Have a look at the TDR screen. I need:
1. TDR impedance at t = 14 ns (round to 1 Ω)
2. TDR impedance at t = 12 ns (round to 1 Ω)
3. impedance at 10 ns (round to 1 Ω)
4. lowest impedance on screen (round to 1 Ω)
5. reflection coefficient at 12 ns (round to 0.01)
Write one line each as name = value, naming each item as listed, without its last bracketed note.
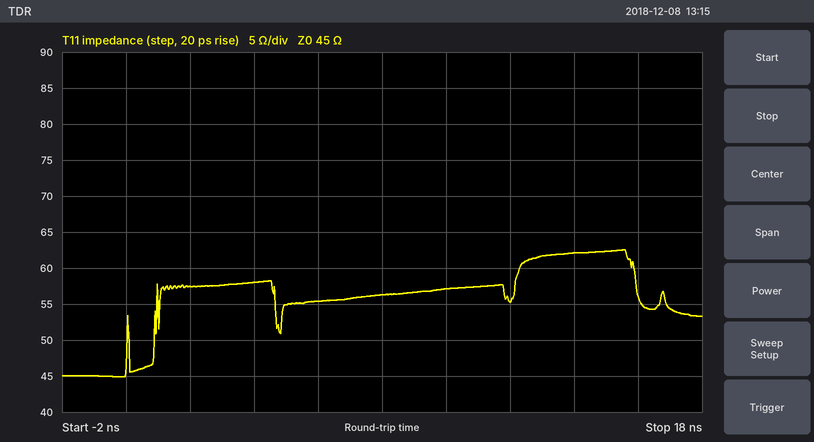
TDR impedance at t = 14 ns = 62 Ω
TDR impedance at t = 12 ns = 55 Ω
impedance at 10 ns = 57 Ω
lowest impedance on screen = 45 Ω
reflection coefficient at 12 ns = +0.10
